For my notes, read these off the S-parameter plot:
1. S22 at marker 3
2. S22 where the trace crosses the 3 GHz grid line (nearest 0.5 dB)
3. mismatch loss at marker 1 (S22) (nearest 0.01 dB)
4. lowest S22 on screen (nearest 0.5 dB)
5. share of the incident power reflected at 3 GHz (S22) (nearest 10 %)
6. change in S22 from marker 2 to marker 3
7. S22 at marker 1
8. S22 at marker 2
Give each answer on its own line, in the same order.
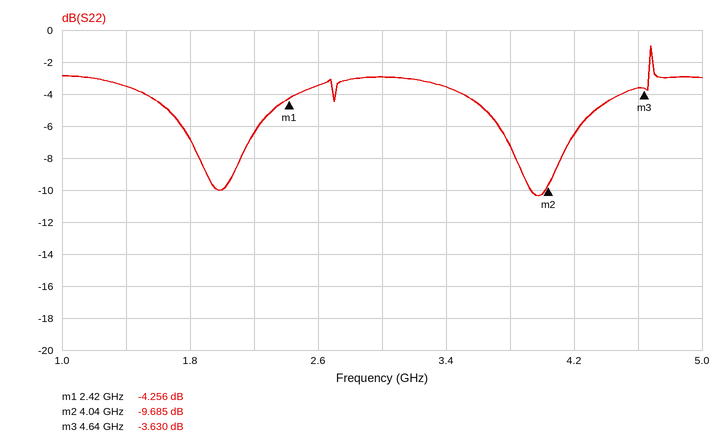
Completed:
-3.630 dB
-3.0 dB
2.04 dB
-10.5 dB
50 %
6.055 dB
-4.256 dB
-9.685 dB
